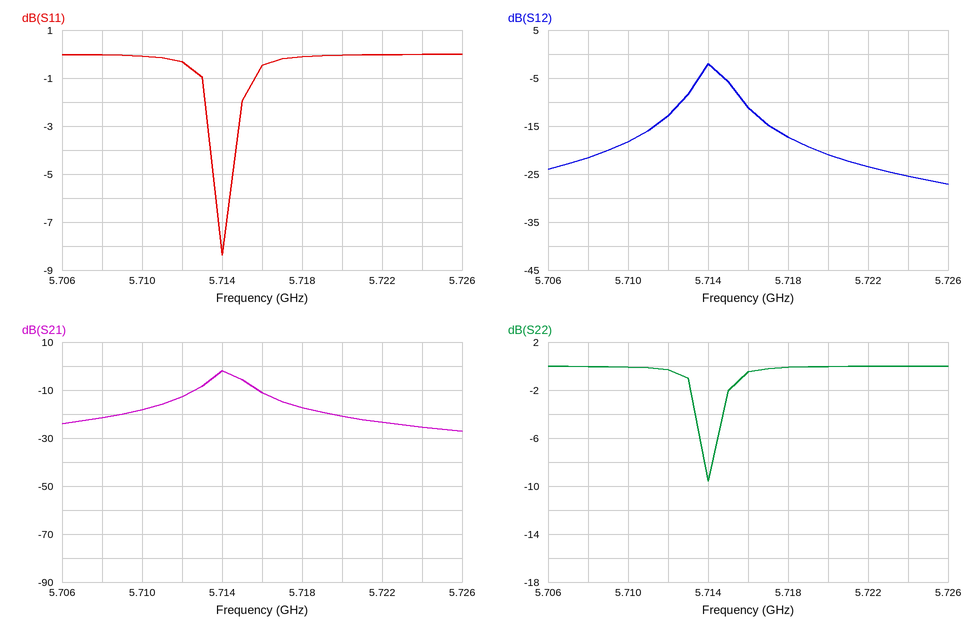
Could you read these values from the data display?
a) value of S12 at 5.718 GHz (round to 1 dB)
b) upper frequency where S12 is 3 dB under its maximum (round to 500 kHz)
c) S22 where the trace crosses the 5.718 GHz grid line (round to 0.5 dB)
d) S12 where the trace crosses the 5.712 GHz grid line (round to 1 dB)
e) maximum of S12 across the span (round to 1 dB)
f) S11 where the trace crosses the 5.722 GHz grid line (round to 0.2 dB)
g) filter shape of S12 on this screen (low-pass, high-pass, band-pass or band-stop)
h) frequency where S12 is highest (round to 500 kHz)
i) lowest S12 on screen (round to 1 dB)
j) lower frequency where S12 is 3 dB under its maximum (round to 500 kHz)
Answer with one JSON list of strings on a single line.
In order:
["-17 dB", "5.7150 GHz", "0.0 dB", "-13 dB", "-2 dB", "0.0 dB", "band-pass", "5.7140 GHz", "-27 dB", "5.7135 GHz"]
